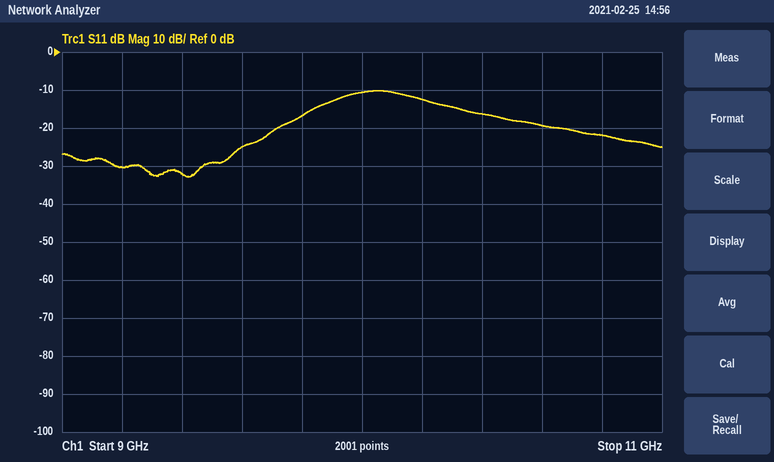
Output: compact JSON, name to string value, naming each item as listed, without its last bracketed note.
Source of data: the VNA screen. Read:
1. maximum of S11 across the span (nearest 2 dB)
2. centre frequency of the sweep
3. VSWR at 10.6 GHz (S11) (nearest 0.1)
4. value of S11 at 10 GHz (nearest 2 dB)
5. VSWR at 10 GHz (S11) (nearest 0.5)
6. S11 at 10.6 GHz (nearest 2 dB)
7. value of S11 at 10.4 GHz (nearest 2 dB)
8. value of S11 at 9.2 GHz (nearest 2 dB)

{"maximum of S11 across the span": "-10 dB", "centre frequency of the sweep": "10 GHz", "VSWR at 10.6 GHz (S11)": "1.2", "value of S11 at 10 GHz": "-10 dB", "VSWR at 10 GHz (S11)": "2.0", "S11 at 10.6 GHz": "-20 dB", "value of S11 at 10.4 GHz": "-16 dB", "value of S11 at 9.2 GHz": "-30 dB"}
